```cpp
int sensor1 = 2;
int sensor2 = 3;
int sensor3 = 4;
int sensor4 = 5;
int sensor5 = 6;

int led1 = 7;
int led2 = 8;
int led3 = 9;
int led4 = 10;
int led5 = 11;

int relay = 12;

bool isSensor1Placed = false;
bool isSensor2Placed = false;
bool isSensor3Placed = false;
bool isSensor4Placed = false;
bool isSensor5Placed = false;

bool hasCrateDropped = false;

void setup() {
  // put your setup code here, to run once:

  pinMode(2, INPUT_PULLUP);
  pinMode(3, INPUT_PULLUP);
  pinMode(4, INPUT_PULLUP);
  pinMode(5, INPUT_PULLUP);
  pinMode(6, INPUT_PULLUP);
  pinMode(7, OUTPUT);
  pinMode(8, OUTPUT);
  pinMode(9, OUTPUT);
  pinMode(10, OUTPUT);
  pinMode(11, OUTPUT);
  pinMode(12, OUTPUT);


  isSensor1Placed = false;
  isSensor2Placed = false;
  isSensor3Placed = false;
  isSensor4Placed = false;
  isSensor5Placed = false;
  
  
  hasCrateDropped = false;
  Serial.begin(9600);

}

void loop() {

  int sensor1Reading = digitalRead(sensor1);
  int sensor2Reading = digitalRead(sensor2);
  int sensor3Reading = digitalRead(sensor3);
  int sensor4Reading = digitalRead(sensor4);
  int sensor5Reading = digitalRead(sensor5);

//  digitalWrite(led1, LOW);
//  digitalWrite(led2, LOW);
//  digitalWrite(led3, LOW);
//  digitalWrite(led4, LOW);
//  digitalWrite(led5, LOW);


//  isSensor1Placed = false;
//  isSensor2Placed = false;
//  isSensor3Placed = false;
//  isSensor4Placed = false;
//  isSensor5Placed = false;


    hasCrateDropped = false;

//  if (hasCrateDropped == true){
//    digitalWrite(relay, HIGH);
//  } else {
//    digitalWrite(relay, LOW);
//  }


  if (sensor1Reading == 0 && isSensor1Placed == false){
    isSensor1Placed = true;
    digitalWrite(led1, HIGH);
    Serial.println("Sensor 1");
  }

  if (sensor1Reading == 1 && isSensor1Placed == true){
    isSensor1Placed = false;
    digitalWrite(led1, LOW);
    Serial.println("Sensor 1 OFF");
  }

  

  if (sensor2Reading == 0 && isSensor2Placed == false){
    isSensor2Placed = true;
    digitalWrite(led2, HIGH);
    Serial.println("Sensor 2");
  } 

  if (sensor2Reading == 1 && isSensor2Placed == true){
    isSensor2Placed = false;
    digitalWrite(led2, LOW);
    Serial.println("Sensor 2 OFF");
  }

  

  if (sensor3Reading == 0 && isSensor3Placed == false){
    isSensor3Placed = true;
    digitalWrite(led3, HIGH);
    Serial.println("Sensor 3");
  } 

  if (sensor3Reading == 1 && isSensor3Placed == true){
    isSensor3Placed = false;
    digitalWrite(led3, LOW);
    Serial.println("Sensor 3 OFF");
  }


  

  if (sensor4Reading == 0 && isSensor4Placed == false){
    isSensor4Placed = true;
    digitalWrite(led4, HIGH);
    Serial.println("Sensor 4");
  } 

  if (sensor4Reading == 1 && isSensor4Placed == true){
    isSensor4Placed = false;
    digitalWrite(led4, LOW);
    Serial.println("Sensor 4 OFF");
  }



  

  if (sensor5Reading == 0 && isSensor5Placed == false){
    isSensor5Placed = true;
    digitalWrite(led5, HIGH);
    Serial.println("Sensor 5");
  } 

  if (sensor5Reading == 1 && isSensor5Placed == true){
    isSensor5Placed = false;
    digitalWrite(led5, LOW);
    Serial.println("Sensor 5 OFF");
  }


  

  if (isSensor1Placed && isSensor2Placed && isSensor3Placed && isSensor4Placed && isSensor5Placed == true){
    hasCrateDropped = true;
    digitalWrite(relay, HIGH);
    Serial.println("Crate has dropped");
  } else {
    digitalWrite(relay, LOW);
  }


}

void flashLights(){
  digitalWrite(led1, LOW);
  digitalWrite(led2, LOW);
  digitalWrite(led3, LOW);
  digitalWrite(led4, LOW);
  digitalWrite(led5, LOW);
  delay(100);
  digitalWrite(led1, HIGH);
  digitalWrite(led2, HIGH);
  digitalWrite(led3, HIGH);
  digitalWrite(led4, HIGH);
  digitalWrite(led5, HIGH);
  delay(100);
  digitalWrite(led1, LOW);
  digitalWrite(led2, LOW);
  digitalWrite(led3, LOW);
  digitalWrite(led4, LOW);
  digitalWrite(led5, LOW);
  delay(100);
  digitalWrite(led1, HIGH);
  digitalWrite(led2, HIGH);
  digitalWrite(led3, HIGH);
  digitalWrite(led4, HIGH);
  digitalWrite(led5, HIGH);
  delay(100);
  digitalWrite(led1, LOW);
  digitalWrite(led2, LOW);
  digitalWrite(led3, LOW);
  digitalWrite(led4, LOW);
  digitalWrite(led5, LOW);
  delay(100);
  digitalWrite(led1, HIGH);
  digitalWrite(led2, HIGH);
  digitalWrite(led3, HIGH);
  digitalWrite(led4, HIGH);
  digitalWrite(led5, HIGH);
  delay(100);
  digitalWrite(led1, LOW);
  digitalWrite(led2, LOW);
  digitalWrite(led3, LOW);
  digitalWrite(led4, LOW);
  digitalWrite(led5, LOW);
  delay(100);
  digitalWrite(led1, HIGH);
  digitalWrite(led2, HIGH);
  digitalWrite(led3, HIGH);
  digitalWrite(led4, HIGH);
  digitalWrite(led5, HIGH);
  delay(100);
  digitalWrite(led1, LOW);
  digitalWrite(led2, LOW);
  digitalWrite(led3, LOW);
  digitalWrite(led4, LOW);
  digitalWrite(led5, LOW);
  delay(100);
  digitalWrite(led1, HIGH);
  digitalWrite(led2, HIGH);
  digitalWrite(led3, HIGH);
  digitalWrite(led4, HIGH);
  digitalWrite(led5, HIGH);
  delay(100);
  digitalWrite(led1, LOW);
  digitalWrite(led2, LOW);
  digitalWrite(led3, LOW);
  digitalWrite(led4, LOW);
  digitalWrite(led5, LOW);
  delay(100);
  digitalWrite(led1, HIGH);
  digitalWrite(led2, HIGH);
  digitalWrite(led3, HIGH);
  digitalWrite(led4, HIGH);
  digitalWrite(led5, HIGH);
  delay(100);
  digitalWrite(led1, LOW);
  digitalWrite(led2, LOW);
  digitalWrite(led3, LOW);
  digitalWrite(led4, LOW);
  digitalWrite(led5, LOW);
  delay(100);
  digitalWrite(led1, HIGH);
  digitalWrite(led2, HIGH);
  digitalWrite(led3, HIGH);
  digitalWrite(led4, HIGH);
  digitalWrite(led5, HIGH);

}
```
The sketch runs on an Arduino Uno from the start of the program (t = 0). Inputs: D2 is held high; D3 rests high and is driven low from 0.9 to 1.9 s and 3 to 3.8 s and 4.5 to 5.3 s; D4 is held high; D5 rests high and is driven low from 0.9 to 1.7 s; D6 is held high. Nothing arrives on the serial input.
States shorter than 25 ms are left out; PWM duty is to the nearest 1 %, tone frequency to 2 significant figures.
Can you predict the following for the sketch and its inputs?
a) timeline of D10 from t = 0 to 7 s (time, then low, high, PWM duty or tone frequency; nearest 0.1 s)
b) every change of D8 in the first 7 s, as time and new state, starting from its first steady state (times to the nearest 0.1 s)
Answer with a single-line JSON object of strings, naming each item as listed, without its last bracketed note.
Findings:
{"timeline of D10 from t = 0 to 7 s": "0 s low; 0.9 s high; 1.7 s low", "every change of D8 in the first 7 s, as time and new state, starting from its first steady state": "0 s low; 0.9 s high; 1.9 s low; 3 s high; 3.8 s low; 4.5 s high; 5.3 s low"}
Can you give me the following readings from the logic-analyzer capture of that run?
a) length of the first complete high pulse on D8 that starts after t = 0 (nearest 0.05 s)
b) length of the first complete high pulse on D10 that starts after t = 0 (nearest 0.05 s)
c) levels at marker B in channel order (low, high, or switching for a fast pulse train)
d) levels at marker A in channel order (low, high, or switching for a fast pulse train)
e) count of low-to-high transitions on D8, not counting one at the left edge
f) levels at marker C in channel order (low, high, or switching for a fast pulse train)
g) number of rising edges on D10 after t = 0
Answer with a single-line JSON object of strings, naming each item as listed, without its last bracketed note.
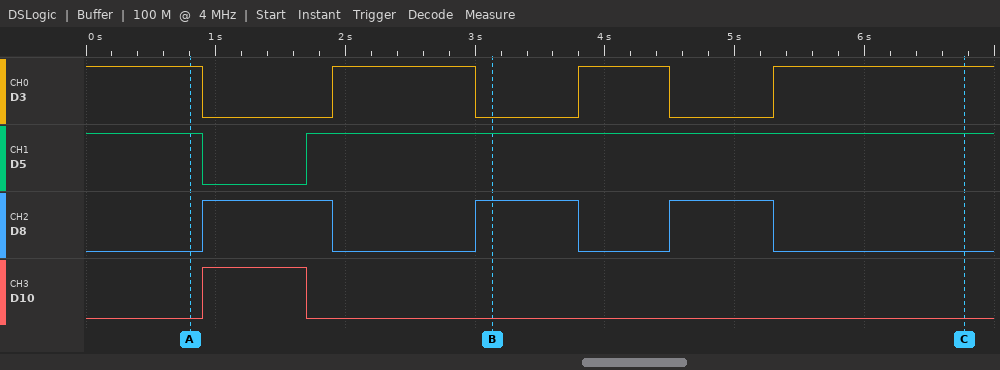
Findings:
{"length of the first complete high pulse on D8 that starts after t = 0": "1.00 s", "length of the first complete high pulse on D10 that starts after t = 0": "0.80 s", "levels at marker B in channel order": "D3 low, D5 high, D8 high, D10 low", "levels at marker A in channel order": "D3 high, D5 high, D8 low, D10 low", "count of low-to-high transitions on D8, not counting one at the left edge": "3", "levels at marker C in channel order": "D3 high, D5 high, D8 low, D10 low", "number of rising edges on D10 after t = 0": "1"}
